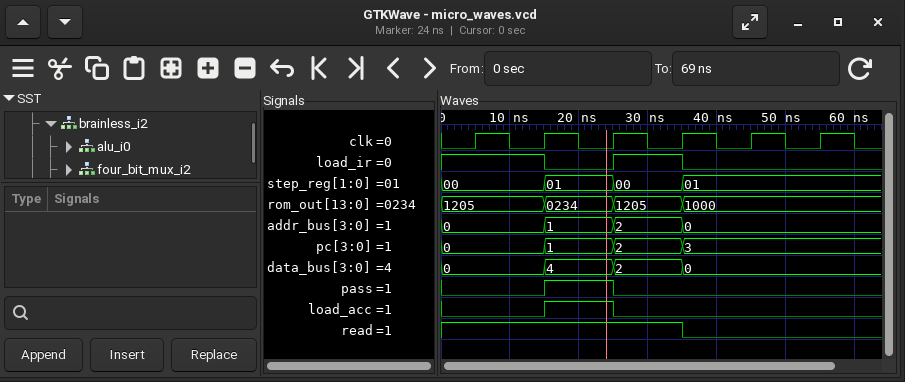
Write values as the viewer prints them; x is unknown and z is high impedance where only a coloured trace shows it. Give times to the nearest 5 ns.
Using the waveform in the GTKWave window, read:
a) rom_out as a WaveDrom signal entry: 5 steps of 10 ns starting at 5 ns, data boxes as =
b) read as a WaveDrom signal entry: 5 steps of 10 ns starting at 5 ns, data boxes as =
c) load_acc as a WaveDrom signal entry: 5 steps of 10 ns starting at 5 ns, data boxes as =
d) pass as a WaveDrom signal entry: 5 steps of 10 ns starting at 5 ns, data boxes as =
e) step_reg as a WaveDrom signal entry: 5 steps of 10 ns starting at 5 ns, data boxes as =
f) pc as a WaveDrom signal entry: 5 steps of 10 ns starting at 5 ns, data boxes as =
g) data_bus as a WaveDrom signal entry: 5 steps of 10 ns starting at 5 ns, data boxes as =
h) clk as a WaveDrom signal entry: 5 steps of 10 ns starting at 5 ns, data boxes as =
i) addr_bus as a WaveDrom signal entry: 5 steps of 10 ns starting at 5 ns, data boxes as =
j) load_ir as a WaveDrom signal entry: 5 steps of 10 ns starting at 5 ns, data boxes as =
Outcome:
{name: 'rom_out', wave: '====.', data: '1205 0234 1205 1000'}
{name: 'read', wave: '1..0.'}
{name: 'load_acc', wave: '010..'}
{name: 'pass', wave: '010..'}
{name: 'step_reg', wave: '====.', data: '00 01 00 01'}
{name: 'pc', wave: '====.', data: '0 1 2 3'}
{name: 'data_bus', wave: '====.', data: '0 4 2 0'}
{name: 'clk', wave: 'p....'}
{name: 'addr_bus', wave: '====.', data: '0 1 2 0'}
{name: 'load_ir', wave: '1010.'}
